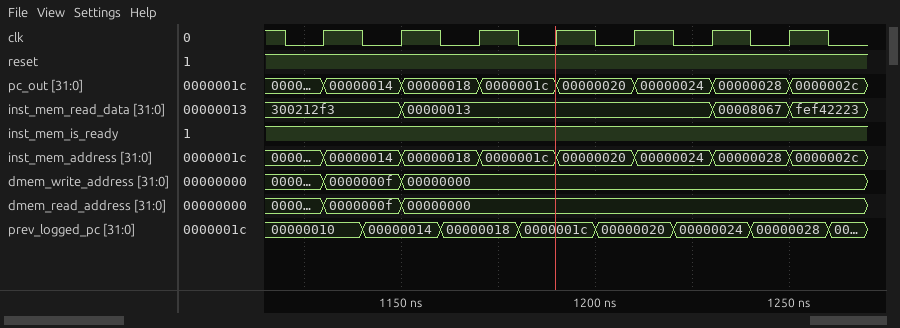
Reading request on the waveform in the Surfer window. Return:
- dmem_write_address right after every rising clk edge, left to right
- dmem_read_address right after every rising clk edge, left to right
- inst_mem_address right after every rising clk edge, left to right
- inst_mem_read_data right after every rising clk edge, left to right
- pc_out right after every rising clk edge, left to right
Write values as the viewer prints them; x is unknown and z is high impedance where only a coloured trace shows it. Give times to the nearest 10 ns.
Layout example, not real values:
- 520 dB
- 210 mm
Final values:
- 0000000f, 00000000, 00000000, 00000000, 00000000, 00000000, 00000000
- 0000000f, 00000000, 00000000, 00000000, 00000000, 00000000, 00000000
- 00000014, 00000018, 0000001c, 00000020, 00000024, 00000028, 0000002c
- 300212f3, 00000013, 00000013, 00000013, 00000013, 00008067, fef42223
- 00000014, 00000018, 0000001c, 00000020, 00000024, 00000028, 0000002c
